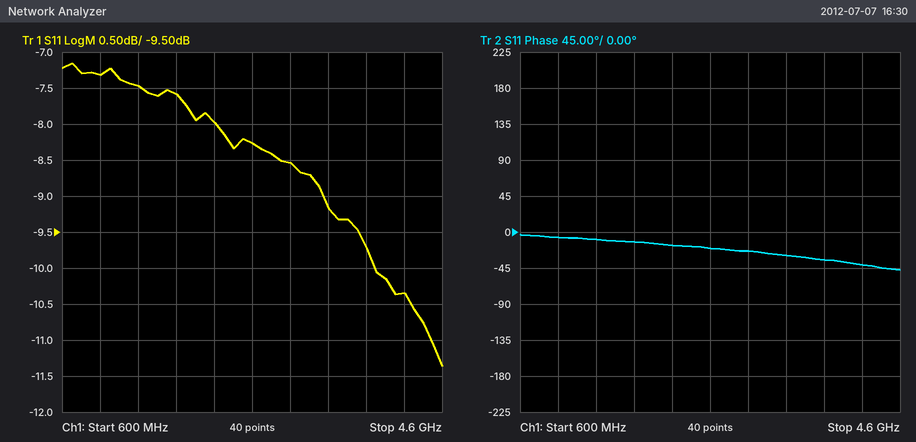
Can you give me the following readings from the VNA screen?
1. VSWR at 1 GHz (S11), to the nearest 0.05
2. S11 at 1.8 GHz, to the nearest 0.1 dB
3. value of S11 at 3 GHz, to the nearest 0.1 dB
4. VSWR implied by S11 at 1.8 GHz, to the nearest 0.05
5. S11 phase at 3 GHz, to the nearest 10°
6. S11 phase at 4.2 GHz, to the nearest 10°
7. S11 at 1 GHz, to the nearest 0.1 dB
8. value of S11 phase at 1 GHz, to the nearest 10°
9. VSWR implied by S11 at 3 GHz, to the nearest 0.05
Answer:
2.50
-7.6 dB
-8.5 dB
2.45
-20°
-40°
-7.3 dB
-10°
2.20
